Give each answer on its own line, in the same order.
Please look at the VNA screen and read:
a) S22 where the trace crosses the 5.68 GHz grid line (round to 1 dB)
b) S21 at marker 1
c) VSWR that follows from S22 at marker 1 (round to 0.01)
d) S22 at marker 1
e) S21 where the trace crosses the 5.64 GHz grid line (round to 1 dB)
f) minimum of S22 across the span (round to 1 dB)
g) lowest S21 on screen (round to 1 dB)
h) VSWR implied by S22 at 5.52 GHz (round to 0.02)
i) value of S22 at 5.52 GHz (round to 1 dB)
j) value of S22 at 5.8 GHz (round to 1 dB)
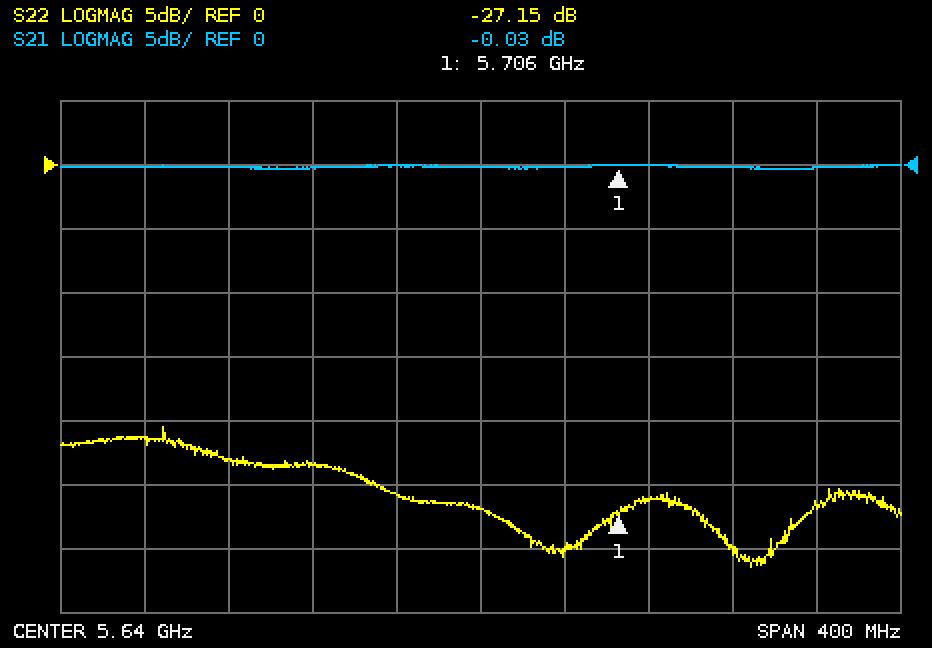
-30 dB
-0.03 dB
1.09
-27.15 dB
0 dB
-31 dB
0 dB
1.16
-23 dB
-27 dB
